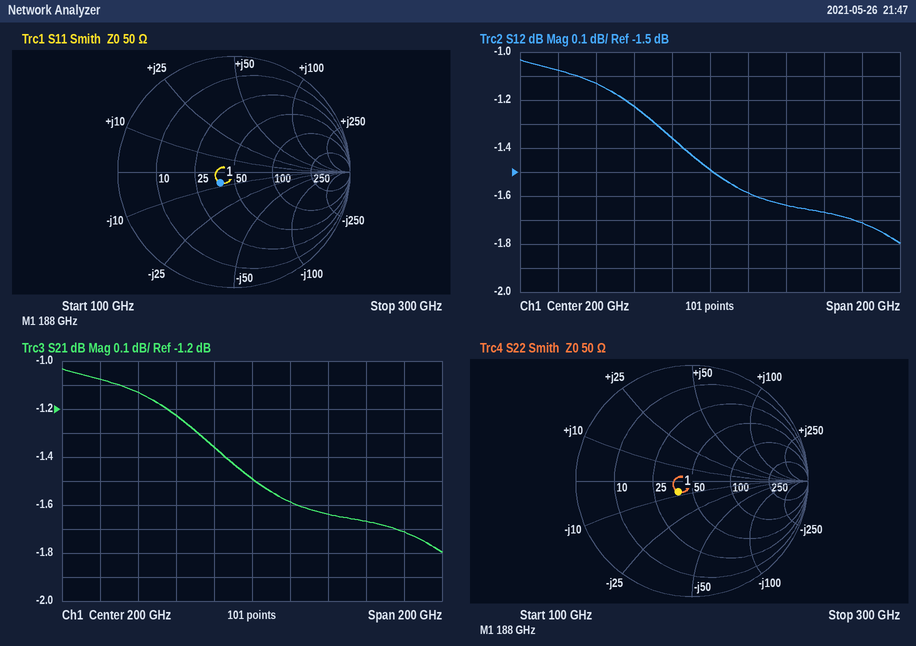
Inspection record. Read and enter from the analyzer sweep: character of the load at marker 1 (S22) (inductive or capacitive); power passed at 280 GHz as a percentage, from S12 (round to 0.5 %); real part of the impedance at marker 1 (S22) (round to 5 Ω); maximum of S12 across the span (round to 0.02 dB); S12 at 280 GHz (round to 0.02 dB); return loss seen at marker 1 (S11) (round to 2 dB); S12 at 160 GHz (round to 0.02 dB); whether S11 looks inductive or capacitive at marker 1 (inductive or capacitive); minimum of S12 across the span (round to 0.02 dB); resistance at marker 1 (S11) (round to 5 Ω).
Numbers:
capacitive
67.5 %
40 Ω
-1.04 dB
-1.72 dB
16 dB
-1.22 dB
capacitive
-1.80 dB
40 Ω
